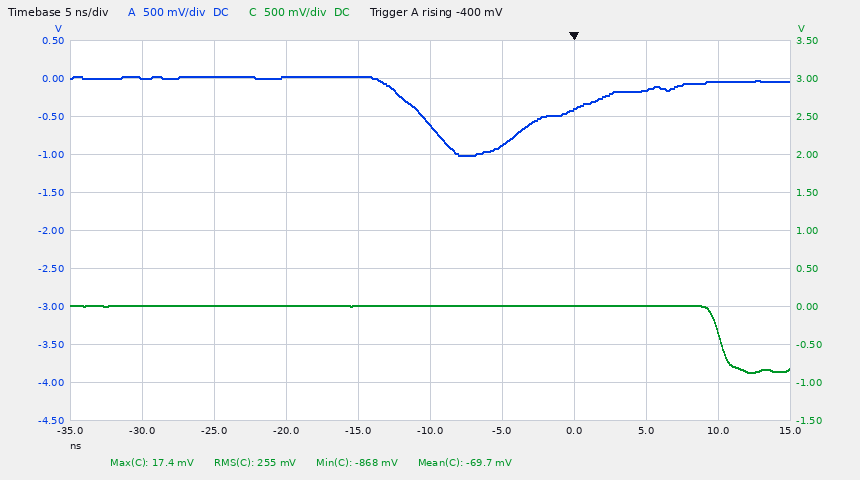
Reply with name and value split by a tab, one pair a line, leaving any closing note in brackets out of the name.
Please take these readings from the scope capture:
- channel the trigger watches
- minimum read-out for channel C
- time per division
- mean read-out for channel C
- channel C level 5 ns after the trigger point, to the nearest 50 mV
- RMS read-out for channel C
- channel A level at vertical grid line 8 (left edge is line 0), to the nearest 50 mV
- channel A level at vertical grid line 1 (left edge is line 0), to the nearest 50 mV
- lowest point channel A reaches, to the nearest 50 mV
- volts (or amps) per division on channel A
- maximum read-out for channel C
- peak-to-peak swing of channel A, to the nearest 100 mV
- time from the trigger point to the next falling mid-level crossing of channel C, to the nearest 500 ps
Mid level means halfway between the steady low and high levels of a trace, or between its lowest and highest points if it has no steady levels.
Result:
channel the trigger watches	channel A
minimum read-out for channel C	-868 mV
time per division	5 ns
mean read-out for channel C	-69.7 mV
channel C level 5 ns after the trigger point, to the nearest 50 mV	0 mV
RMS read-out for channel C	255 mV
channel A level at vertical grid line 8 (left edge is line 0), to the nearest 50 mV	-150 mV
channel A level at vertical grid line 1 (left edge is line 0), to the nearest 50 mV	0 mV
lowest point channel A reaches, to the nearest 50 mV	-1.00 V
volts (or amps) per division on channel A	500 mV
maximum read-out for channel C	17.4 mV
peak-to-peak swing of channel A, to the nearest 100 mV	1.00 V
time from the trigger point to the next falling mid-level crossing of channel C, to the nearest 500 ps	10.0 ns
